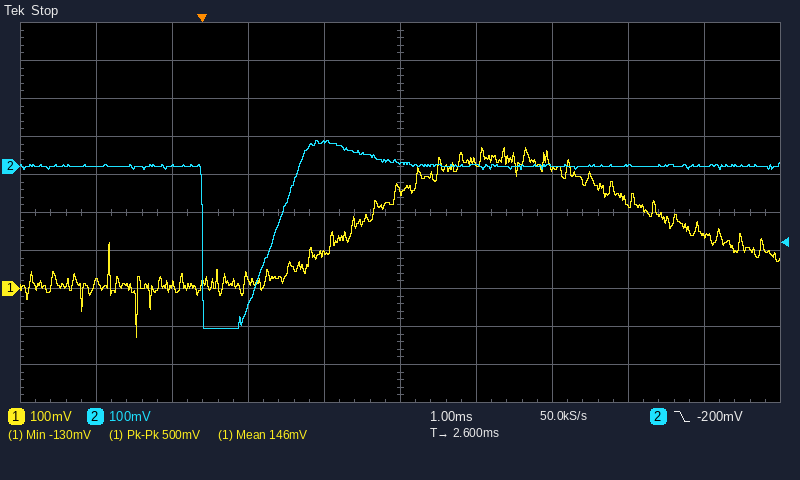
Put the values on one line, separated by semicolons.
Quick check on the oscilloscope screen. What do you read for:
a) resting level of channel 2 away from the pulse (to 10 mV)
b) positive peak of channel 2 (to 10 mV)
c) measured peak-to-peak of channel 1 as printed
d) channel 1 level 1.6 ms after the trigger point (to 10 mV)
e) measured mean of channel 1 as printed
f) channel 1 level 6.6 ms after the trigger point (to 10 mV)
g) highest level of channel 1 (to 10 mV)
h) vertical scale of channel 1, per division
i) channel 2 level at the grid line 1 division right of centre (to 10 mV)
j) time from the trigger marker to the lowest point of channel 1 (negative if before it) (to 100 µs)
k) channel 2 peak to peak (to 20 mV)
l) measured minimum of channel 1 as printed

0 mV; 70 mV; 500 mV; 90 mV; 146 mV; 140 mV; 370 mV; 100 mV; 0 mV; -900 µs; 500 mV; -130 mV
